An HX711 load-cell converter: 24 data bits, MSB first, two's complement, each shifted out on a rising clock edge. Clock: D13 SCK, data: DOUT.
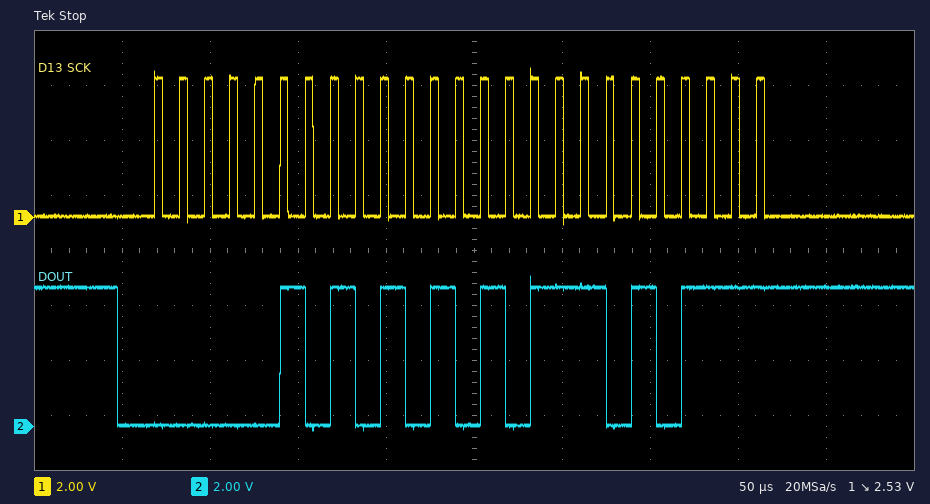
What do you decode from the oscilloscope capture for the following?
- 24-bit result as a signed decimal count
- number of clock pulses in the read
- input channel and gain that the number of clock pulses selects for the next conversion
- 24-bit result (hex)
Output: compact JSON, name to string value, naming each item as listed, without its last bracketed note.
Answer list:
{"24-bit result as a signed decimal count": "349655", "number of clock pulses in the read": "25", "input channel and gain that the number of clock pulses selects for the next conversion": "channel A, gain 128", "24-bit result": "0x0555D7"}
